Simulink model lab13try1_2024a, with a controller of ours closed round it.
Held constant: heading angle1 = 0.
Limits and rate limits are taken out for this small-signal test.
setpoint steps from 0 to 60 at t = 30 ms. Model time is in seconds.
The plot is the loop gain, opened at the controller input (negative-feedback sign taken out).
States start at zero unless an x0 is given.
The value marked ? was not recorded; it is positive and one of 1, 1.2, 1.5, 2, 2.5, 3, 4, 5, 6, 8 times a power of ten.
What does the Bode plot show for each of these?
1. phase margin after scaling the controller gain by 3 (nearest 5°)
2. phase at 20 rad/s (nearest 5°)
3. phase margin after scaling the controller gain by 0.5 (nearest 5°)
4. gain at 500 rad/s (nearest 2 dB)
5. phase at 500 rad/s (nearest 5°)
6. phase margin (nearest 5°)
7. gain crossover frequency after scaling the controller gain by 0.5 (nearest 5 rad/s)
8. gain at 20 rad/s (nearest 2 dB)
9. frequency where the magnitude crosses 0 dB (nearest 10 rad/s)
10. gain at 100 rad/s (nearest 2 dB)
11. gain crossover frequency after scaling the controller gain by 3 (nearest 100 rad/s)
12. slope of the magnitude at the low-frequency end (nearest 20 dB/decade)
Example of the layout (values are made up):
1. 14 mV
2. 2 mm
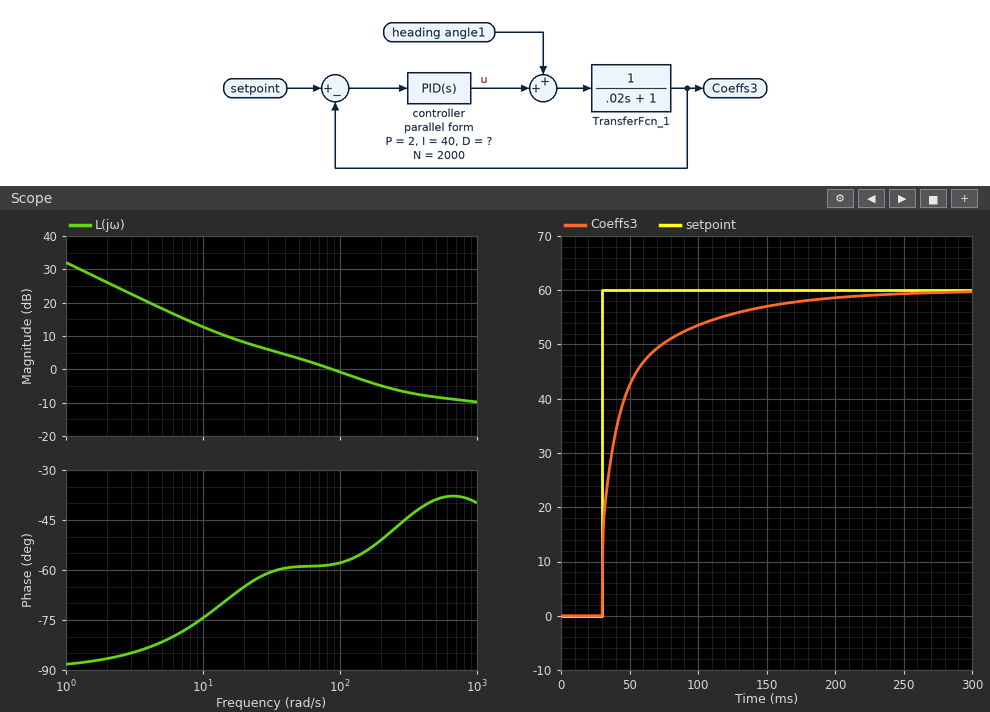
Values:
1. 140°
2. -65°
3. 120°
4. -8 dB
5. -40°
6. 120°
7. 30 rad/s
8. 8 dB
9. 90 rad/s
10. 0 dB
11. 900 rad/s
12. -20 dB/decade
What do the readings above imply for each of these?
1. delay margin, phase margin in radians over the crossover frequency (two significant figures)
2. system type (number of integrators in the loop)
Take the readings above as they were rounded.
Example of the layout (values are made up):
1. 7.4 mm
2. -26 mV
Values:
1. 0.023 s
2. 1
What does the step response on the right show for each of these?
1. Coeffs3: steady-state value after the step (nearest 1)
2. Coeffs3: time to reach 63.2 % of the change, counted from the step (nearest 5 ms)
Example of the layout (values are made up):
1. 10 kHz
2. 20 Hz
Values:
1. 60
2. 15 ms
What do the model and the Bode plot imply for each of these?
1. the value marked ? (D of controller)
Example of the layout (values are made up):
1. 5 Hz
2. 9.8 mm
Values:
1. 0.006
